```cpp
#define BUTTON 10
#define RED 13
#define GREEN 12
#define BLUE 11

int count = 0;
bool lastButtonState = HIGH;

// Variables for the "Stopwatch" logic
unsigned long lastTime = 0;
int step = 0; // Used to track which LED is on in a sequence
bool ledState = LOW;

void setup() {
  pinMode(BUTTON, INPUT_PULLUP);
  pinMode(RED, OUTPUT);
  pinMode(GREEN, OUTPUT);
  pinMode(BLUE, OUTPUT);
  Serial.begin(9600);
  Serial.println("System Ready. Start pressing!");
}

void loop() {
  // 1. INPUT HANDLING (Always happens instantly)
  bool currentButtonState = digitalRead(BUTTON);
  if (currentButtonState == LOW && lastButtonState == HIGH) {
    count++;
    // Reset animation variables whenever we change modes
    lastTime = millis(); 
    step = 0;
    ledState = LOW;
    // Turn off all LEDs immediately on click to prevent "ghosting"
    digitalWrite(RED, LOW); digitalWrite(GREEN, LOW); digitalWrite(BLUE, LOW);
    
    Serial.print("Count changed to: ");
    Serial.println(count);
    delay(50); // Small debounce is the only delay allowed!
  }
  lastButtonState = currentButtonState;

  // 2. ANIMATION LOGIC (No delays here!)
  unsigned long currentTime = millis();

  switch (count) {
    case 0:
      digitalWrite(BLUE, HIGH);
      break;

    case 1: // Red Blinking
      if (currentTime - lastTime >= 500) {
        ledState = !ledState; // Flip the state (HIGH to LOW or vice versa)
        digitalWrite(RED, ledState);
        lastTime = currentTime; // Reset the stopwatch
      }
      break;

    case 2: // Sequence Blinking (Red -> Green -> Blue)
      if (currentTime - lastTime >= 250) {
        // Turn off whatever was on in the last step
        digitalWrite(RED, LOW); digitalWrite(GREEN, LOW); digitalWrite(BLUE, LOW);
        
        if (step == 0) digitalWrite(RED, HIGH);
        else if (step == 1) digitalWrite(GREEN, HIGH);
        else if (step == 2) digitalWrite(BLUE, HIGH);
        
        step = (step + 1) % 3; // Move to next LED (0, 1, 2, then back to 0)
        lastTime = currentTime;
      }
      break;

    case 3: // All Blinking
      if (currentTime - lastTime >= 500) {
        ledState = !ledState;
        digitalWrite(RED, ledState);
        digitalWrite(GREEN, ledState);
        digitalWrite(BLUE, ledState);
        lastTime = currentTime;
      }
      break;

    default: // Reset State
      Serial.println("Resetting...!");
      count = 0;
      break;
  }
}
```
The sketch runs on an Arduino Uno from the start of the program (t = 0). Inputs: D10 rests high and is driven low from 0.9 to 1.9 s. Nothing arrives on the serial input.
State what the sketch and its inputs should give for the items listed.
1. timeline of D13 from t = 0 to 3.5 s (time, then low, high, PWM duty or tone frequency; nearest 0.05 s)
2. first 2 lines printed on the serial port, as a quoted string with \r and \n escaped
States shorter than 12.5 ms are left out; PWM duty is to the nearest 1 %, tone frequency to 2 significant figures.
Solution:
0 s low; 1.4 s high; 1.9 s low; 2.4 s high; 2.9 s low; 3.4 s high
"System Ready. Start pressing!\r\nCount changed to: 1\r\n"
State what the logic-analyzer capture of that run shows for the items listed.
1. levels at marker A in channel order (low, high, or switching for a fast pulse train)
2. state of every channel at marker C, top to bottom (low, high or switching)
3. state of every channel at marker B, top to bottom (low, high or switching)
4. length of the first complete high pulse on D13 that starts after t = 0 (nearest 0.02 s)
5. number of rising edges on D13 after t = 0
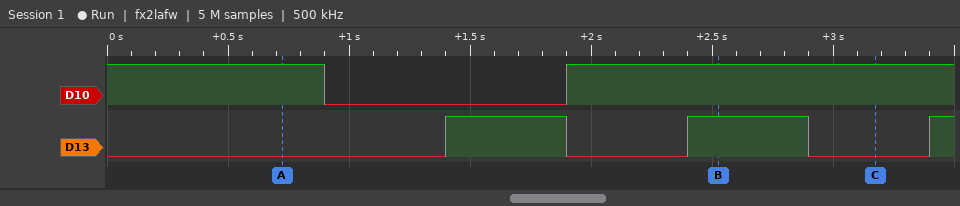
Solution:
D10 high, D13 low
D10 high, D13 low
D10 high, D13 high
0.50 s
3
